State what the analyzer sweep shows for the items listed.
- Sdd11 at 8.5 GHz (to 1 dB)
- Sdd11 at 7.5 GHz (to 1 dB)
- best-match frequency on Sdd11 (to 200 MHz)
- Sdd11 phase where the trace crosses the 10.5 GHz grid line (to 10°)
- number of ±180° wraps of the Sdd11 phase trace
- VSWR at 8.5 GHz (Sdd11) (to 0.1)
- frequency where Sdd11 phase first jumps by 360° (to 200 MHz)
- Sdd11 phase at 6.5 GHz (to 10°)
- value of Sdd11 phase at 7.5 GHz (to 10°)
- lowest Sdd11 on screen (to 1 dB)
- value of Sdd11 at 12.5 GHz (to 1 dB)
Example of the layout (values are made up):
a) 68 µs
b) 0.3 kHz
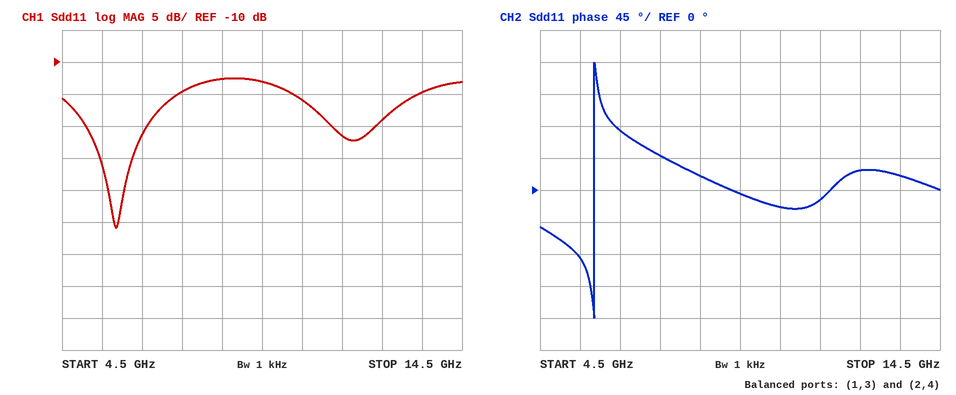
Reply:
a) -13 dB
b) -15 dB
c) 5.8 GHz
d) -20°
e) 1
f) 1.6
g) 5.8 GHz
h) 80°
i) 50°
j) -36 dB
k) -19 dB
